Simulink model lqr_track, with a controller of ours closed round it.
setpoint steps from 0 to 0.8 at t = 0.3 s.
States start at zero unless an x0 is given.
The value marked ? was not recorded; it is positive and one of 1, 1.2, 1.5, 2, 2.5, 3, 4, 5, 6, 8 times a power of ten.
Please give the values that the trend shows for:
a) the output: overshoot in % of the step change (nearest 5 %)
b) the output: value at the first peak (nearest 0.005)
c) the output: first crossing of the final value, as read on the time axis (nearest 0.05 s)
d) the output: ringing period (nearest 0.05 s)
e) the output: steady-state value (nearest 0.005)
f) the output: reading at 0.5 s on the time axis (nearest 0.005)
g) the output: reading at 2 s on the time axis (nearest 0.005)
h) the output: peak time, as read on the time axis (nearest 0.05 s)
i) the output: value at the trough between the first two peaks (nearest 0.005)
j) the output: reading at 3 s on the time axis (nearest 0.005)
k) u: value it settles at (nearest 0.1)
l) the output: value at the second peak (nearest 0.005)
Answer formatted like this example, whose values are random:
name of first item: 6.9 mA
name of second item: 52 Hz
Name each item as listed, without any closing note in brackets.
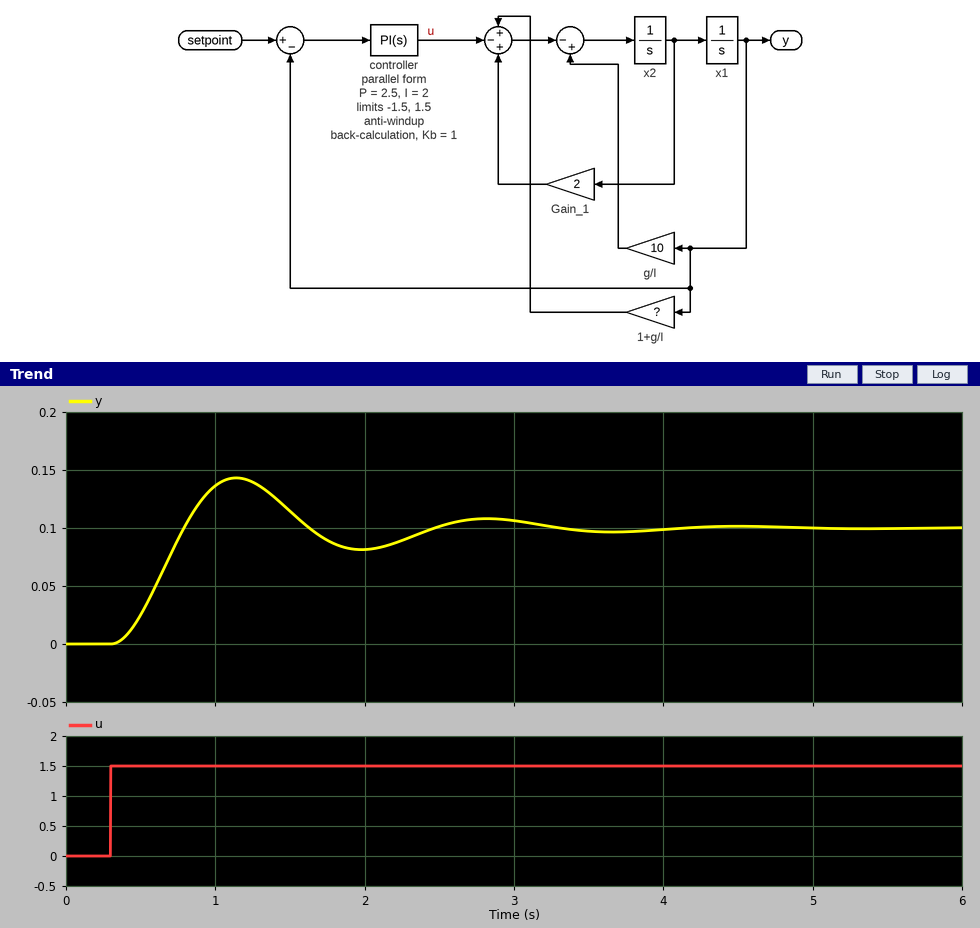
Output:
the output: overshoot in % of the step change: 45 %
the output: value at the first peak: 0.145
the output: first crossing of the final value, as read on the time axis: 0.80 s
the output: ringing period: 1.70 s
the output: steady-state value: 0.100
the output: reading at 0.5 s on the time axis: 0.025
the output: reading at 2 s on the time axis: 0.080
the output: peak time, as read on the time axis: 1.15 s
the output: value at the trough between the first two peaks: 0.080
the output: reading at 3 s on the time axis: 0.105
u: value it settles at: 1.5
the output: value at the second peak: 0.110
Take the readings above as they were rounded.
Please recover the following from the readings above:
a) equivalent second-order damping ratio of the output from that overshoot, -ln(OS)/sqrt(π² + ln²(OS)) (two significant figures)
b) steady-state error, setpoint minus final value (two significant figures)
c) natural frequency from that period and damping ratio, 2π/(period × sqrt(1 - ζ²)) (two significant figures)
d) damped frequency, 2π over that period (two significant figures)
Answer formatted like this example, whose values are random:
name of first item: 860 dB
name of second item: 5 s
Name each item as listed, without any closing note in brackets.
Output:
equivalent second-order damping ratio of the output from that overshoot, -ln(OS)/sqrt(π² + ln²(OS)): 0.25
steady-state error, setpoint minus final value: 0.70
natural frequency from that period and damping ratio, 2π/(period × sqrt(1 - ζ²)): 3.8 rad/s
damped frequency, 2π over that period: 3.7 rad/s
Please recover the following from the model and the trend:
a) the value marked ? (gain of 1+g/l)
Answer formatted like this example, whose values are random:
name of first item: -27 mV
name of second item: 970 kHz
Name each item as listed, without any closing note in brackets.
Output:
the value marked ?: 25
